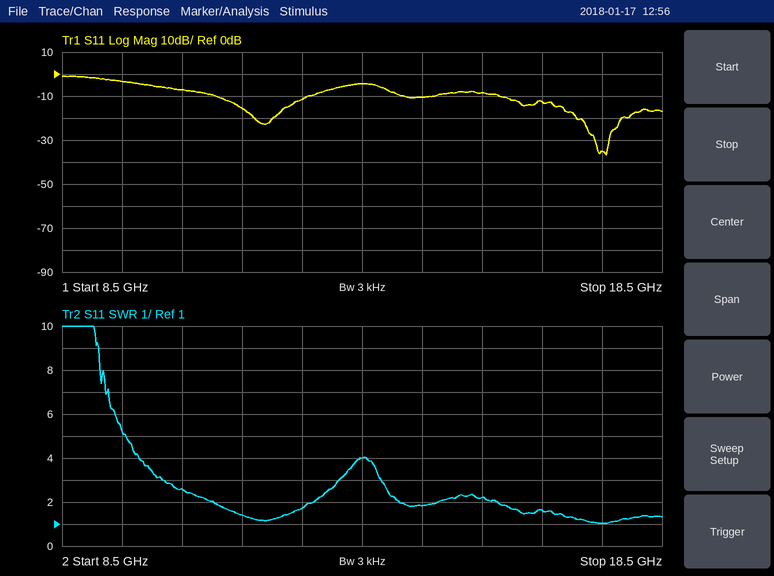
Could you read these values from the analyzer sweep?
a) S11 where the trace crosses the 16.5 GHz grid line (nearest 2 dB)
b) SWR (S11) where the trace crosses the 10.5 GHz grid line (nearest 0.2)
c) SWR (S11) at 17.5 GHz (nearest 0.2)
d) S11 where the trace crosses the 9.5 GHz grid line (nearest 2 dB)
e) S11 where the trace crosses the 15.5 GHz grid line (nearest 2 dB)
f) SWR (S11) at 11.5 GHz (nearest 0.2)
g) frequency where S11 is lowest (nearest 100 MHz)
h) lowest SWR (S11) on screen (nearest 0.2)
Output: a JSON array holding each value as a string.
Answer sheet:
["-12 dB", "2.6", "1.0", "-4 dB", "-8 dB", "1.4", "17.6 GHz", "1.0"]
